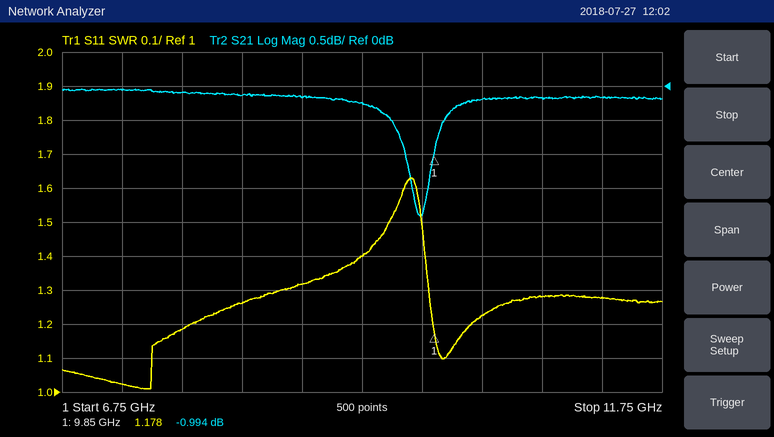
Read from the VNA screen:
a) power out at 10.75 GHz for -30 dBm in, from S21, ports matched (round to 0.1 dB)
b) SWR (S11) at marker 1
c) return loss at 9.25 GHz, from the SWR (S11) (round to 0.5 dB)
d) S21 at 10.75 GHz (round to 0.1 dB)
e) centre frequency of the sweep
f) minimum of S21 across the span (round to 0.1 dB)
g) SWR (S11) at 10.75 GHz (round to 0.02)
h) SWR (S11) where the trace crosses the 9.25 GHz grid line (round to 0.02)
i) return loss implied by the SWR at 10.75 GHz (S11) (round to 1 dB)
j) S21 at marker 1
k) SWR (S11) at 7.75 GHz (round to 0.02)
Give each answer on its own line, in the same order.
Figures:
-30.2 dBm
1.178
15.5 dB
-0.2 dB
9.25 GHz
-1.9 dB
1.28
1.40
18 dB
-0.994 dB
1.18
